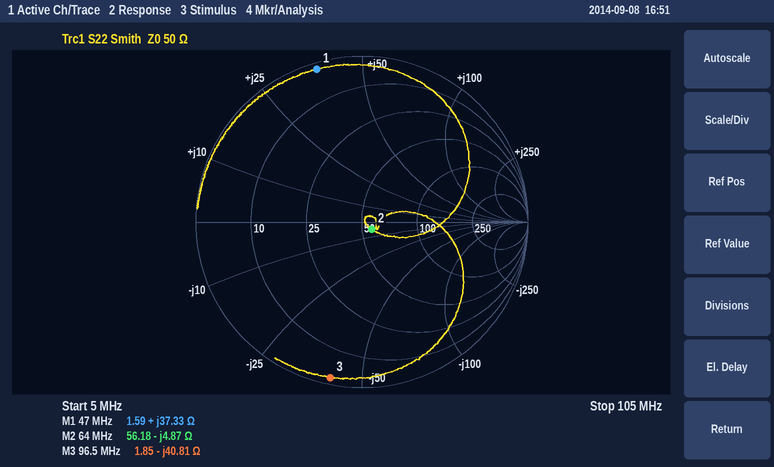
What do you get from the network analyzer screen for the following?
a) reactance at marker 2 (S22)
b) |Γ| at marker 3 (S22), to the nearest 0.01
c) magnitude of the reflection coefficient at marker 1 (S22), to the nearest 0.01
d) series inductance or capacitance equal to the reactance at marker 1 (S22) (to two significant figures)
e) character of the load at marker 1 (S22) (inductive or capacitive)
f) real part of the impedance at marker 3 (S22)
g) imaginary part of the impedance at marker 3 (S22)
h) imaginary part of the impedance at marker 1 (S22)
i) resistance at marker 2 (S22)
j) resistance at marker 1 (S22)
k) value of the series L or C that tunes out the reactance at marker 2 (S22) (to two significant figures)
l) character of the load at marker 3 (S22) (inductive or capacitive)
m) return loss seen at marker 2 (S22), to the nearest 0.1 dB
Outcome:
-4.87 Ω
0.96
0.96
130 nH
inductive
1.85 Ω
-40.81 Ω
+37.33 Ω
56.18 Ω
1.59 Ω
12 nH
capacitive
22.6 dB
